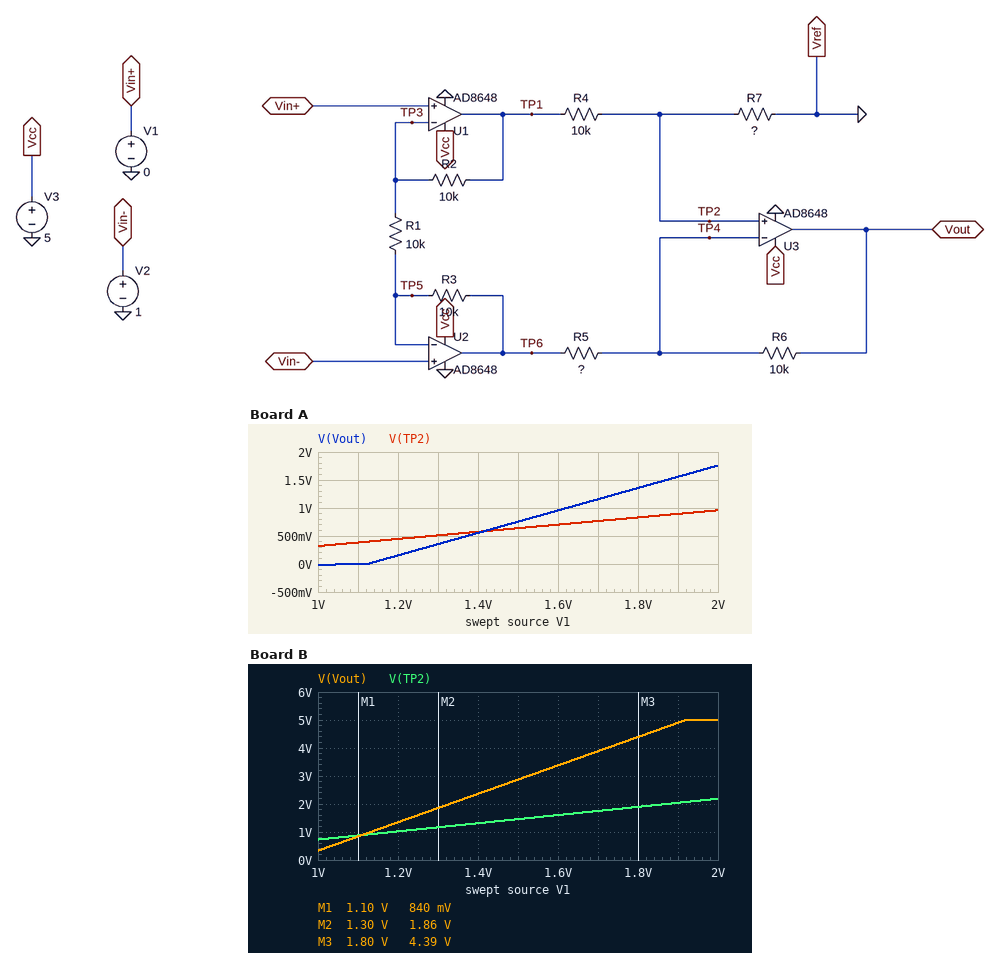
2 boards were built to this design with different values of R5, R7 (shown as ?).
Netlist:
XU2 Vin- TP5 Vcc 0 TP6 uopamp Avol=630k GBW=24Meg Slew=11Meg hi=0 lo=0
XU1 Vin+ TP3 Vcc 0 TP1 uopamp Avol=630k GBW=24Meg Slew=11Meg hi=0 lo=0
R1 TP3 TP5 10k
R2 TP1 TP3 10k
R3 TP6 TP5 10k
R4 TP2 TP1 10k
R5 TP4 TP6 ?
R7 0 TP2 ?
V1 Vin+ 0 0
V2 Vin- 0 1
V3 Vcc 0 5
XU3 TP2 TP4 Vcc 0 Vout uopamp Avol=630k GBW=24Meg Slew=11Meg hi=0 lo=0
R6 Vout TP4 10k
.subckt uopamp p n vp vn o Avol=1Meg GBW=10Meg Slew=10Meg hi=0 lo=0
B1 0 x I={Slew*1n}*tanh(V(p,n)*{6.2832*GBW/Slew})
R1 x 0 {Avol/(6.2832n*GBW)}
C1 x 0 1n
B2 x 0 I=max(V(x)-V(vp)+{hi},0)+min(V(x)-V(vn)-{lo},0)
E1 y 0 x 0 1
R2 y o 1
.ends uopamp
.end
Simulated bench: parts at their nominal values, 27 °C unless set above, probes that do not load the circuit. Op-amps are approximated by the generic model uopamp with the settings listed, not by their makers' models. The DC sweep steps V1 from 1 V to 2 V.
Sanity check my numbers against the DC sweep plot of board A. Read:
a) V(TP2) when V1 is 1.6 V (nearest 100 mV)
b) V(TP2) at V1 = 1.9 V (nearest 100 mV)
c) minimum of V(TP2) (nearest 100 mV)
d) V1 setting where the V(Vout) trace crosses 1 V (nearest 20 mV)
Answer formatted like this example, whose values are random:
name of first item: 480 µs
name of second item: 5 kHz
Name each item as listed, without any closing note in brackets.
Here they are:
V(TP2) when V1 is 1.6 V: 700 mV
V(TP2) at V1 = 1.9 V: 900 mV
minimum of V(TP2): 300 mV
V1 setting where the V(Vout) trace crosses 1 V: 1.62 V
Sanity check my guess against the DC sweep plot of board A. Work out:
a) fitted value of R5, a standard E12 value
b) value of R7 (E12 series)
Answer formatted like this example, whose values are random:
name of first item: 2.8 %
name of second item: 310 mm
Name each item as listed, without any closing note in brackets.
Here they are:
fitted value of R5, a standard E12 value: 12 kΩ
value of R7: 4.7 kΩ
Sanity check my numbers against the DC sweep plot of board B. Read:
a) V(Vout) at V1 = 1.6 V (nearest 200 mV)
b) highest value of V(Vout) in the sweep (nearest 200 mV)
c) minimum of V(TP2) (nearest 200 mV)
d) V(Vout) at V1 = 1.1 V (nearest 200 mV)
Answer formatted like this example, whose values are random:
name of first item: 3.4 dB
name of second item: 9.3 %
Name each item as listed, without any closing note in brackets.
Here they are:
V(Vout) at V1 = 1.6 V: 3.4 V
highest value of V(Vout) in the sweep: 5.0 V
minimum of V(TP2): 800 mV
V(Vout) at V1 = 1.1 V: 800 mV
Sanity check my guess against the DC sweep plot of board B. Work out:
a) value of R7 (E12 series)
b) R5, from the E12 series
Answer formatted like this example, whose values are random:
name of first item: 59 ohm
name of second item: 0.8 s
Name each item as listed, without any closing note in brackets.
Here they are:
value of R7: 27 kΩ
R5, from the E12 series: 6.8 kΩ
